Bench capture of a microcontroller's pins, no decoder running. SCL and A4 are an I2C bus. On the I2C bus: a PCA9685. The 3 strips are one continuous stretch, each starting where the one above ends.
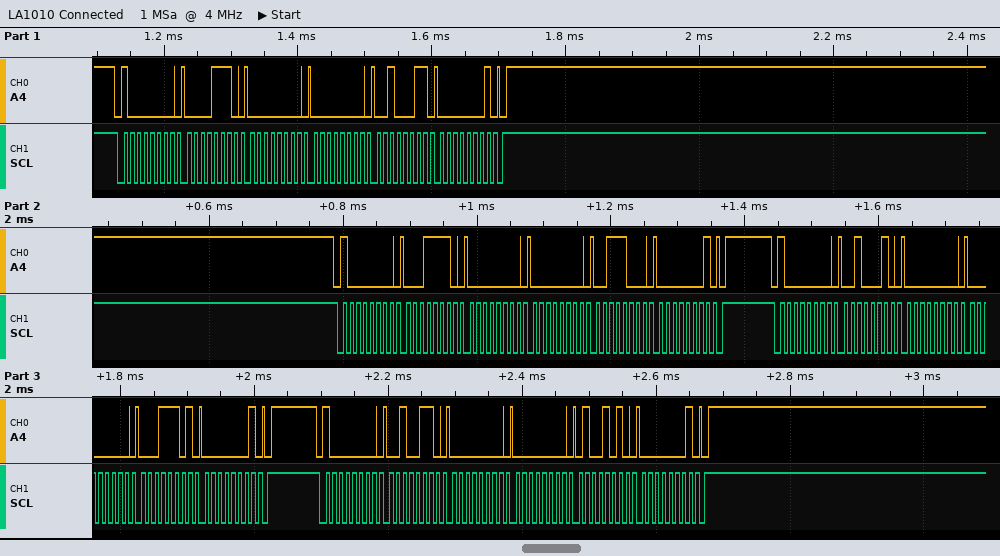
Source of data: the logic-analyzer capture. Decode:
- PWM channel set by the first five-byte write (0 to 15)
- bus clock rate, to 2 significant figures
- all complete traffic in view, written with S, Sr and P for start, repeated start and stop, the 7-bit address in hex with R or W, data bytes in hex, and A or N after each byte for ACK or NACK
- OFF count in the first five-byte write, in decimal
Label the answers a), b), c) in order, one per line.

a) 2
b) 100 kHz
c) S 40W A 0E A 00 A 00 A 23 A 01 A P S 40W A 1E A 00 A 00 A 38 A 01 A P S 40W A 22 A 00 A 00 A 1D A 01 A P S 40W A 26 A 00 A 00 A 4A A 01 A P
d) 291
